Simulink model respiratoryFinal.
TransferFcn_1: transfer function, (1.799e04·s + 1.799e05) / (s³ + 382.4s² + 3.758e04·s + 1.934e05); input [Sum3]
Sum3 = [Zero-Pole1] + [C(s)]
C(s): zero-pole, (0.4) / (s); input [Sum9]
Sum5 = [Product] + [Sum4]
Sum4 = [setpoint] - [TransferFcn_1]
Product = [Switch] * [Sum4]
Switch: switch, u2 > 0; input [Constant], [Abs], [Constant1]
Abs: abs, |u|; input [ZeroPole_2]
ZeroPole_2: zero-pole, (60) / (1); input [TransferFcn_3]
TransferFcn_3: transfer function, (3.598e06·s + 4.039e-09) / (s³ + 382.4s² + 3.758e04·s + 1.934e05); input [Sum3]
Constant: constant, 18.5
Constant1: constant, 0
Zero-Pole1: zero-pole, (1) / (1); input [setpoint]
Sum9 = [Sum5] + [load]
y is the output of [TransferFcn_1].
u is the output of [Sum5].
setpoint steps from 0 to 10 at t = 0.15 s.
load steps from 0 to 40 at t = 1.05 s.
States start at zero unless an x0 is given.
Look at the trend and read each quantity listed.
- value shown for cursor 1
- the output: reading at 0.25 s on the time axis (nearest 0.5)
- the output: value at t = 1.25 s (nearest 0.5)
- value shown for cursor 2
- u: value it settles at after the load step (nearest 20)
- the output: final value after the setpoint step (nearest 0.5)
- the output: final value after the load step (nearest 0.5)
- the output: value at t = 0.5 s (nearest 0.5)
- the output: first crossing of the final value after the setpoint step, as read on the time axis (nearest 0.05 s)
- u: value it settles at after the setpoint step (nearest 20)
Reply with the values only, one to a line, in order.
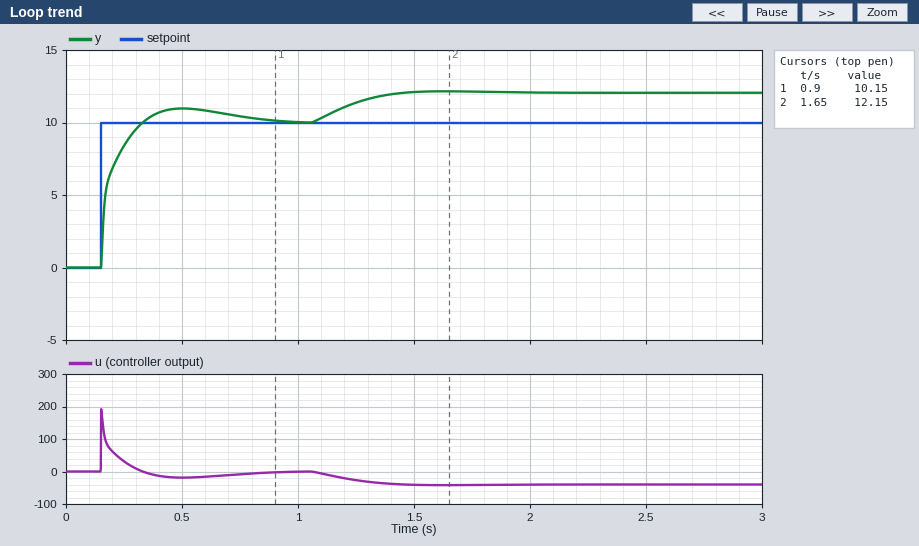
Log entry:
10.15
8.5
11.5
12.15
-40
10.0
12.0
11.0
0.35 s
0
